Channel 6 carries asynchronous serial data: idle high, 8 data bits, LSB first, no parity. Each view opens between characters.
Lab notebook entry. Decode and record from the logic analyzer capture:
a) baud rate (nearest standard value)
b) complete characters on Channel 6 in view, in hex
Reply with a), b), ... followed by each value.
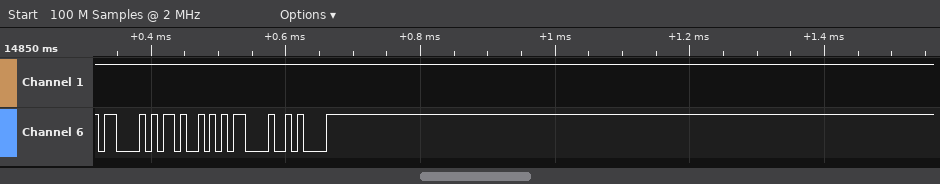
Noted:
a) 115200 baud
b) 43, 4B, 0D, 0A
